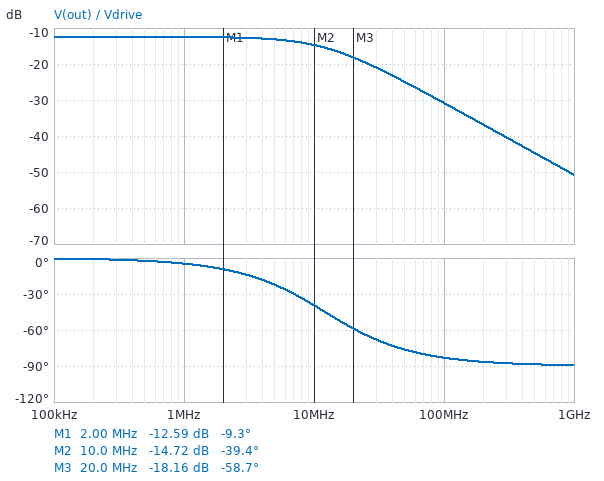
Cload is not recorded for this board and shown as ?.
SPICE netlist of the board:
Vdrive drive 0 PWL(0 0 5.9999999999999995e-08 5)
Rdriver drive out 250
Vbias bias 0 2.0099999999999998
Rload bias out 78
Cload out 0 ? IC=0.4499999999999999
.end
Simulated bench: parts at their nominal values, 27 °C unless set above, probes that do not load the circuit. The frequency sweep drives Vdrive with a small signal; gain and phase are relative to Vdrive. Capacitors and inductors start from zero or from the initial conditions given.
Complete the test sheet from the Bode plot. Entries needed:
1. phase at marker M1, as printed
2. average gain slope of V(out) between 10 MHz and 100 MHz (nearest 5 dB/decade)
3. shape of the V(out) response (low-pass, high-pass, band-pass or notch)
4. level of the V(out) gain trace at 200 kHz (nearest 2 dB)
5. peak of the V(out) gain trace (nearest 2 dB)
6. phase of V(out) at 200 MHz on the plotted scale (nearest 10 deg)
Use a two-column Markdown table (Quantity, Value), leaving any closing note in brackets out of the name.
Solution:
| Quantity | Value |
|---|---|
| phase at marker M1, as printed | -9.3 deg |
| average gain slope of V(out) between 10 MHz and 100 MHz | -15 dB/decade |
| shape of the V(out) response | low-pass |
| level of the V(out) gain trace at 200 kHz | -12 dB |
| peak of the V(out) gain trace | -12 dB |
| phase of V(out) at 200 MHz on the plotted scale | -90 deg |
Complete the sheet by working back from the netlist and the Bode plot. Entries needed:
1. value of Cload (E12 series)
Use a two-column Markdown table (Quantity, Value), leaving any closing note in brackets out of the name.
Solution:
| Quantity | Value |
|---|---|
| value of Cload | 220 pF |
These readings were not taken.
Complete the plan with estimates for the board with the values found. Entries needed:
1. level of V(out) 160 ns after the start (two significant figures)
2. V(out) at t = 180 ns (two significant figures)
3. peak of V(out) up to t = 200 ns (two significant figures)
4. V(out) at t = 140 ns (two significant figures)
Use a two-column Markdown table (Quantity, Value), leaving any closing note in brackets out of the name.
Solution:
| Quantity | Value |
|---|---|
| level of V(out) 160 ns after the start | 2.7 V |
| V(out) at t = 180 ns | 2.7 V |
| peak of V(out) up to t = 200 ns | 2.7 V |
| V(out) at t = 140 ns | 2.7 V |
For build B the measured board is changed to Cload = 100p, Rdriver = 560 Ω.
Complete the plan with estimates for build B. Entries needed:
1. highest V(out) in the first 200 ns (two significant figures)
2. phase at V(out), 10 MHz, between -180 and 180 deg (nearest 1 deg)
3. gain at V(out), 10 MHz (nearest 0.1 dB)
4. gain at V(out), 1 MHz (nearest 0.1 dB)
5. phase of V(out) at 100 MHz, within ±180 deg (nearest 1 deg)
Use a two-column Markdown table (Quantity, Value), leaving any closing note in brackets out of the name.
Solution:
| Quantity | Value |
|---|---|
| highest V(out) in the first 200 ns | 2.4 V |
| phase at V(out), 10 MHz, between -180 and 180 deg | -23 deg |
| gain at V(out), 10 MHz | -19.0 dB |
| gain at V(out), 1 MHz | -18.3 dB |
| phase of V(out) at 100 MHz, within ±180 deg | -77 deg |
